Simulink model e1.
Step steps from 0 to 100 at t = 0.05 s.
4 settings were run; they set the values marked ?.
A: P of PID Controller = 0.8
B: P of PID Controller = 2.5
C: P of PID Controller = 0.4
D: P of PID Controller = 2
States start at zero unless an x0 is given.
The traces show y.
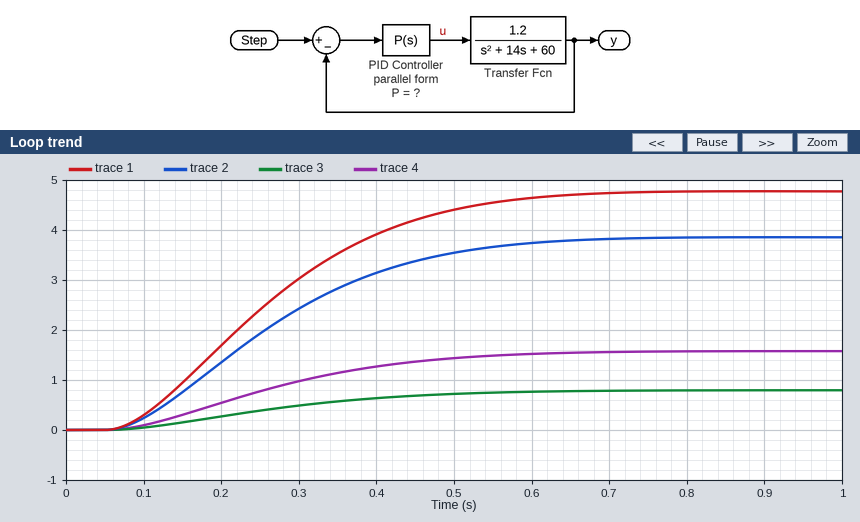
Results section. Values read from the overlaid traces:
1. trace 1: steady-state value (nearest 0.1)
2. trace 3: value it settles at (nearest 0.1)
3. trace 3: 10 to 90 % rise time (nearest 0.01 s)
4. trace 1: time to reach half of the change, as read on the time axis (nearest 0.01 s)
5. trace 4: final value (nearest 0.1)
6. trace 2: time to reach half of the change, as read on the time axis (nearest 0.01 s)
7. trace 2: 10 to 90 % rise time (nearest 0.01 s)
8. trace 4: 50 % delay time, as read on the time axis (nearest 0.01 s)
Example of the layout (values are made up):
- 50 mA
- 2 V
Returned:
- 4.8
- 0.8
- 0.37 s
- 0.25 s
- 1.6
- 0.25 s
- 0.36 s
- 0.25 s
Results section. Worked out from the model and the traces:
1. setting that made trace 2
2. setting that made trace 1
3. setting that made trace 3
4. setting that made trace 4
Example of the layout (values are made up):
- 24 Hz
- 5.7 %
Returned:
- D
- B
- C
- A
